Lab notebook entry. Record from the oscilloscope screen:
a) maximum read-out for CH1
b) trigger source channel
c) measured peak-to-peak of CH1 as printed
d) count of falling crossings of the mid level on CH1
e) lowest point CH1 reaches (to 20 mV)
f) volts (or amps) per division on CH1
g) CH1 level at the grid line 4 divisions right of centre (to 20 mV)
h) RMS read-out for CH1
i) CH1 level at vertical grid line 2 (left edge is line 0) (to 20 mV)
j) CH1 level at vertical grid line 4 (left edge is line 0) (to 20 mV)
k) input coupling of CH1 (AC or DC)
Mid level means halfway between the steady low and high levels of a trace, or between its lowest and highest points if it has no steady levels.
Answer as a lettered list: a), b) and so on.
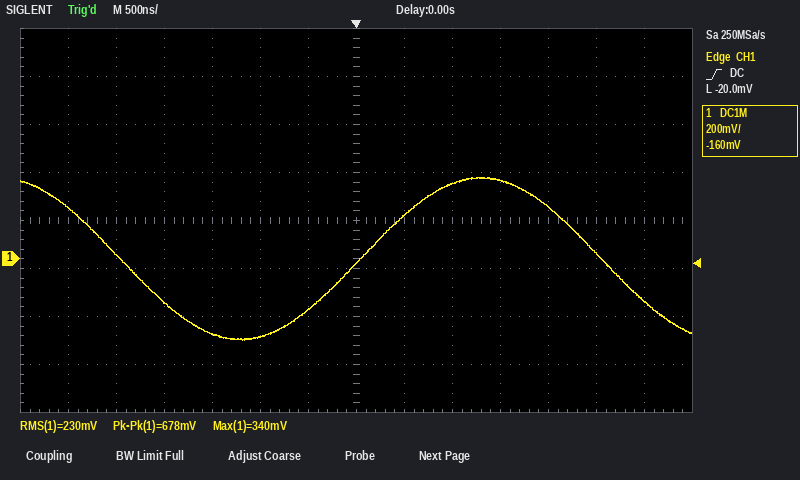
a) 340 mV
b) CH1
c) 678 mV
d) 2
e) -340 mV
f) 200 mV
g) 220 mV
h) 230 mV
i) 20 mV
j) -320 mV
k) DC
